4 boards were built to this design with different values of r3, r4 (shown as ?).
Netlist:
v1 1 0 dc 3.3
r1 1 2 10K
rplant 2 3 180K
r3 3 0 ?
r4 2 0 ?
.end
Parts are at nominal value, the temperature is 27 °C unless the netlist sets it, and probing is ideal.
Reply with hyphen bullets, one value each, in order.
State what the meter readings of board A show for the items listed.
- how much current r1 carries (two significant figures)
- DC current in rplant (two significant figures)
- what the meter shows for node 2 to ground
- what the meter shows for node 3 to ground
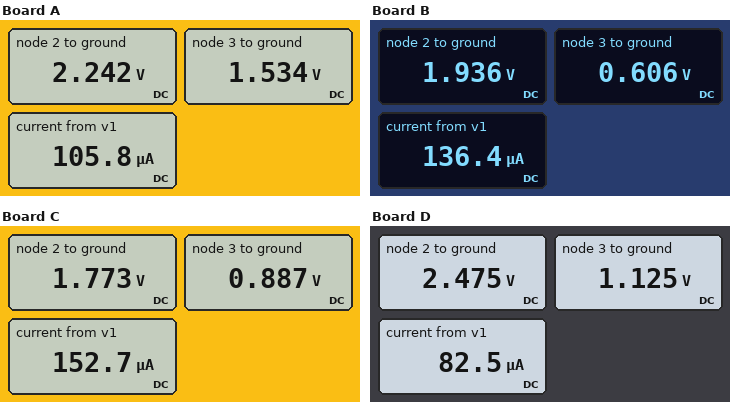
- 110 µA
- 3.9 µA
- 2.242 V
- 1.534 V
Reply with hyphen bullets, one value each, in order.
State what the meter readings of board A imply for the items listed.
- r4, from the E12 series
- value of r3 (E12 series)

- 22 kΩ
- 390 kΩ
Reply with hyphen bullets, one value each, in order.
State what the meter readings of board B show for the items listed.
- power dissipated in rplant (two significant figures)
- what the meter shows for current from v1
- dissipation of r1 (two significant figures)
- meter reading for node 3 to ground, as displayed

- 9.8 µW
- 136.4 µA
- 190 µW
- 0.606 V
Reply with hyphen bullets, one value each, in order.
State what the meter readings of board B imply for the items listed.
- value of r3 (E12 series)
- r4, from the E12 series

- 82 kΩ
- 15 kΩ
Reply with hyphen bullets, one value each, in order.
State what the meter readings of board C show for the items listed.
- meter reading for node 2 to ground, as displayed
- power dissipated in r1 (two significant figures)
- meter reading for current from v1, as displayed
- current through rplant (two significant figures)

- 1.773 V
- 230 µW
- 152.7 µA
- 4.9 µA
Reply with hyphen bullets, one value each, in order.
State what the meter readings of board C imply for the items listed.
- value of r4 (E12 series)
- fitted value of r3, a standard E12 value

- 12 kΩ
- 180 kΩ
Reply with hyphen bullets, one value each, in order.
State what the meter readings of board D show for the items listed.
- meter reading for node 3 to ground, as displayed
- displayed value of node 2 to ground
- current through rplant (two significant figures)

- 1.125 V
- 2.475 V
- 7.5 µA
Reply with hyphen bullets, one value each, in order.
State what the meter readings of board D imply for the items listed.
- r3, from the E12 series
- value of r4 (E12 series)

- 150 kΩ
- 33 kΩ
